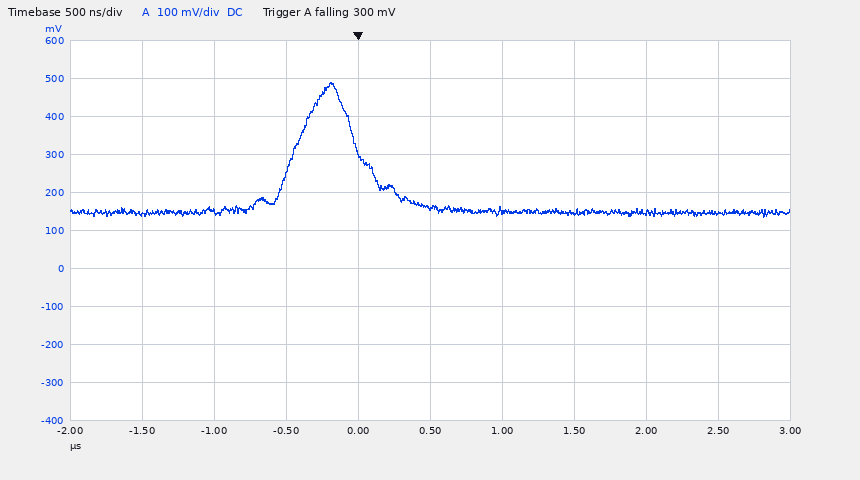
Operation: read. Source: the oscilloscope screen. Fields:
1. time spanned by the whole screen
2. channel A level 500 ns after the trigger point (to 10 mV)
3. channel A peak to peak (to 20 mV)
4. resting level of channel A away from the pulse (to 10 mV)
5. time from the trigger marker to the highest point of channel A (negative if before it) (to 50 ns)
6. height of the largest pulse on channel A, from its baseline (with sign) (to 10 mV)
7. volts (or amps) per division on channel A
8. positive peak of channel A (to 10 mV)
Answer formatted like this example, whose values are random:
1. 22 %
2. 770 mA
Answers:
1. 5 µs
2. 160 mV
3. 360 mV
4. 150 mV
5. -200 ns
6. +340 mV
7. 100 mV
8. 490 mV
